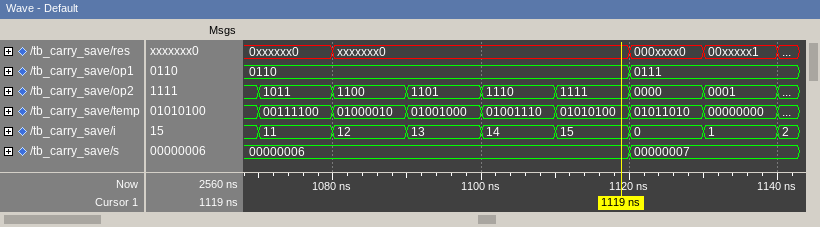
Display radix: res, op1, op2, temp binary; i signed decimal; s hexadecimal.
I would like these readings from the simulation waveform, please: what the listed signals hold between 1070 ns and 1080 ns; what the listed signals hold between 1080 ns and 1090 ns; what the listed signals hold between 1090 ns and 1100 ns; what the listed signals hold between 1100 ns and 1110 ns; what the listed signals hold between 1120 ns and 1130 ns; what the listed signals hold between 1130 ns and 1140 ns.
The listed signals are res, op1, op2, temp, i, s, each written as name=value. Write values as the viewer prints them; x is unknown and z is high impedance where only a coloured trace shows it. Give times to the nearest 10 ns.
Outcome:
res=0xxxxxx0, op1=0110, op2=1011, temp=00111100, i=11, s=00000006
res=xxxxxxx0, op1=0110, op2=1100, temp=01000010, i=12, s=00000006
res=xxxxxxx0, op1=0110, op2=1101, temp=01001000, i=13, s=00000006
res=xxxxxxx0, op1=0110, op2=1110, temp=01001110, i=14, s=00000006
res=000xxxx0, op1=0111, op2=0000, temp=01011010, i=0, s=00000007
res=00xxxxx1, op1=0111, op2=0001, temp=00000000, i=1, s=00000007
